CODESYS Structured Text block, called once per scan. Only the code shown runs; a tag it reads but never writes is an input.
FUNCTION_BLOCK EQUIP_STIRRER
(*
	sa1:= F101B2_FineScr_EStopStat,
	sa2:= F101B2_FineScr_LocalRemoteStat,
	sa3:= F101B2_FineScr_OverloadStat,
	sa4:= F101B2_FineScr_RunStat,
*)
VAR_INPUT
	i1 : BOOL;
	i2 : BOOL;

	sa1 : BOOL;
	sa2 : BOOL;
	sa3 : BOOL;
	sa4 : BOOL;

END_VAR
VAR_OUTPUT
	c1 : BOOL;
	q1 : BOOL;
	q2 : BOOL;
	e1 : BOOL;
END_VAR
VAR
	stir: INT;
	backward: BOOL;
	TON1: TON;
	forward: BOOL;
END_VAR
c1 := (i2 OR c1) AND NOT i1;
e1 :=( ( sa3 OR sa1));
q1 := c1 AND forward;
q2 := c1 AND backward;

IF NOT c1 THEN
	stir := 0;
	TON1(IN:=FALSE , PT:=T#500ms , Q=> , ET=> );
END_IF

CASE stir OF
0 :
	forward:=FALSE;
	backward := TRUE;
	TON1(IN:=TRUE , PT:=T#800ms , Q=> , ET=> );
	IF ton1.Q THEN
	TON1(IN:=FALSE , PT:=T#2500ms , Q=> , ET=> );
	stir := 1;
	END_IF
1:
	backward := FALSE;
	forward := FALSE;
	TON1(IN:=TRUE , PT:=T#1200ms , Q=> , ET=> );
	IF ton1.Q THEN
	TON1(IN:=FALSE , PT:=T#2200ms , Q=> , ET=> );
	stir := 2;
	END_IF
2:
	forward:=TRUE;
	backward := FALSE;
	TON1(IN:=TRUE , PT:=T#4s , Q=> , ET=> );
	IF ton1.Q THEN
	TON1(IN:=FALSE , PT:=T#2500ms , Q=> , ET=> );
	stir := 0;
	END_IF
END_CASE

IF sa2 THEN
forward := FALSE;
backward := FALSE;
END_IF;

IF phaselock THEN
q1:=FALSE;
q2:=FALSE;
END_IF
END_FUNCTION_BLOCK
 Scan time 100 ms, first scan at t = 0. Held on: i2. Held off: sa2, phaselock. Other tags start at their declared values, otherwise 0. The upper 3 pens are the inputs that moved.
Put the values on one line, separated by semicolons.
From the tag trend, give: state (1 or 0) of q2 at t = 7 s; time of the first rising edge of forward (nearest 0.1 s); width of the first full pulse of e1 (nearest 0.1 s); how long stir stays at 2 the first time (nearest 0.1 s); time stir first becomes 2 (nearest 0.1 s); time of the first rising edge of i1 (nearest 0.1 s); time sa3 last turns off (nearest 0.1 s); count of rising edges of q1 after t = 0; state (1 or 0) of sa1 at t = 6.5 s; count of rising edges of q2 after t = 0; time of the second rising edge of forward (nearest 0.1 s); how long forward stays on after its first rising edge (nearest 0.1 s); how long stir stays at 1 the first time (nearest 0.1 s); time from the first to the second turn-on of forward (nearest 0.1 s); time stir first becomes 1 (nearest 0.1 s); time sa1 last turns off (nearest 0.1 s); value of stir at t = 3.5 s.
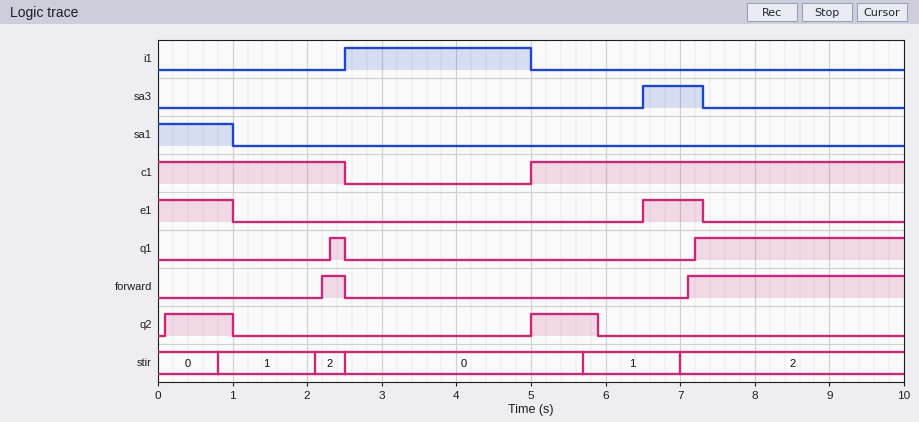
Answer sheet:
0; 2.2 s; 0.8 s; 0.4 s; 2.1 s; 2.5 s; 7.3 s; 2; 0; 2; 7.1 s; 0.3 s; 1.3 s; 4.9 s; 0.8 s; 1.0 s; 0
